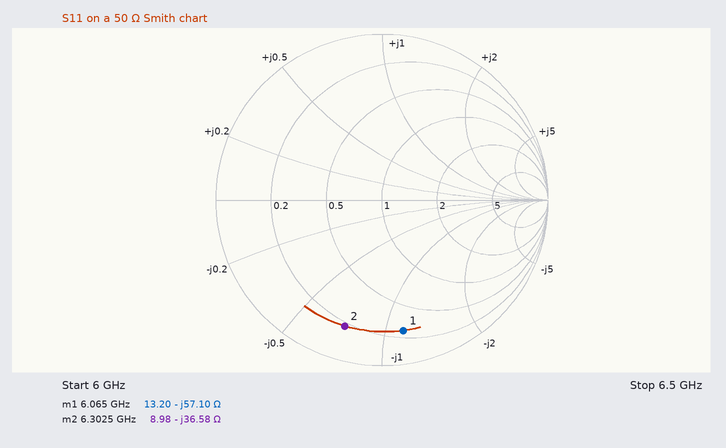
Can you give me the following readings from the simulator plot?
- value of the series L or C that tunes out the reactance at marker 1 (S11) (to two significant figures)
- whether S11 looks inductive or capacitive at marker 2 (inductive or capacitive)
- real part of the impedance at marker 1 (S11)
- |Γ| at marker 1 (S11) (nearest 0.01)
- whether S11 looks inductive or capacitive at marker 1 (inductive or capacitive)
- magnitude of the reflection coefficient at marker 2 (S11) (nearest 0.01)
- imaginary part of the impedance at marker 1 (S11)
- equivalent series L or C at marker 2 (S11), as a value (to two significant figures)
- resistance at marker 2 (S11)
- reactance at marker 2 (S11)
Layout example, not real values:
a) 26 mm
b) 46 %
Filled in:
a) 1.5 nH
b) capacitive
c) 13.20 Ω
d) 0.80
e) capacitive
f) 0.79
g) -57.10 Ω
h) 690 fF
i) 8.98 Ω
j) -36.58 Ω
